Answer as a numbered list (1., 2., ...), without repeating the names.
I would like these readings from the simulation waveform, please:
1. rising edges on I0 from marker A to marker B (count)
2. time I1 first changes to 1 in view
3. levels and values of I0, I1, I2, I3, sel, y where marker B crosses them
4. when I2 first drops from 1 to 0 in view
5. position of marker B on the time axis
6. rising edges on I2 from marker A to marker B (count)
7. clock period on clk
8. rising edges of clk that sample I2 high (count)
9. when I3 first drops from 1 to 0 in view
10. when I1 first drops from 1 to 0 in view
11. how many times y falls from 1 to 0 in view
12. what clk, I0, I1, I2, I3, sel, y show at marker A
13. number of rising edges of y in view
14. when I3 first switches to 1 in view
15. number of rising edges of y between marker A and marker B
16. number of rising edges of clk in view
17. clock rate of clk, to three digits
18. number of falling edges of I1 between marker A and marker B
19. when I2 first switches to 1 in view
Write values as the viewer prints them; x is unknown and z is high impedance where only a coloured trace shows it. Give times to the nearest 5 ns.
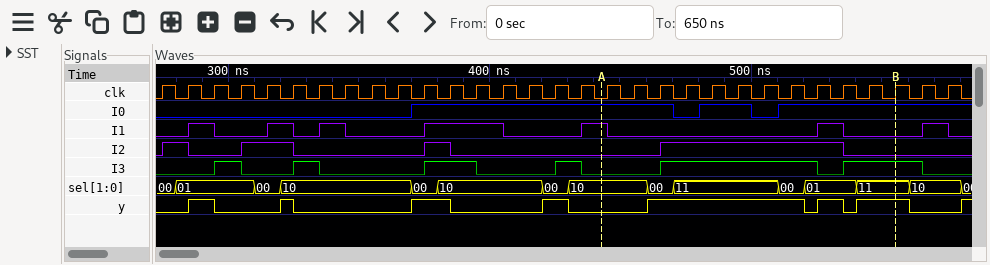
1. 2
2. 285 ns
3. I0=1, I1=0, I2=0, I3=1, sel=11, y=1
4. 285 ns
5. 555 ns
6. 1
7. 10 ns
8. 11
9. 305 ns
10. 295 ns
11. 7
12. clk=0, I0=1, I1=1, I2=0, I3=0, sel=10, y=0
13. 8
14. 295 ns
15. 3
16. 31
17. 100 MHz
18. 2
19. 275 ns
